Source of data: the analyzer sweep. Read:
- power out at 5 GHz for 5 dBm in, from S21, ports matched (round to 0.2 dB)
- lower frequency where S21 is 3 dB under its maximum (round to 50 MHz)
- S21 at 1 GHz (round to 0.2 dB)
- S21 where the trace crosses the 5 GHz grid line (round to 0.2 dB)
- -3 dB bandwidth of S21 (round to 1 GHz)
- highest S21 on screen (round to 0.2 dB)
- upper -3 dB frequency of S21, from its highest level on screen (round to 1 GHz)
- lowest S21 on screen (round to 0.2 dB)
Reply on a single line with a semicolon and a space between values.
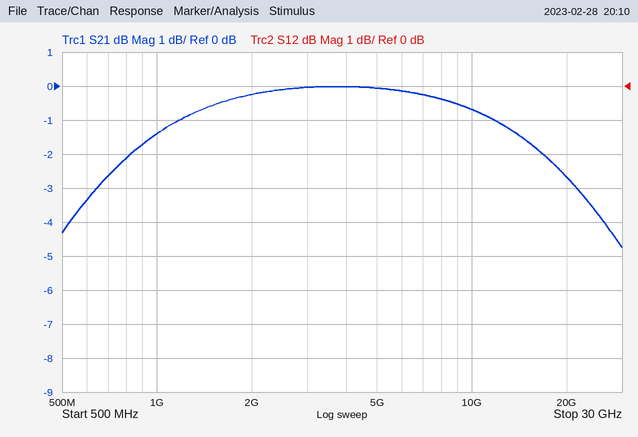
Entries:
5.0 dBm; 650 MHz; -1.4 dB; 0.0 dB; 21 GHz; 0.0 dB; 22 GHz; -4.8 dB
